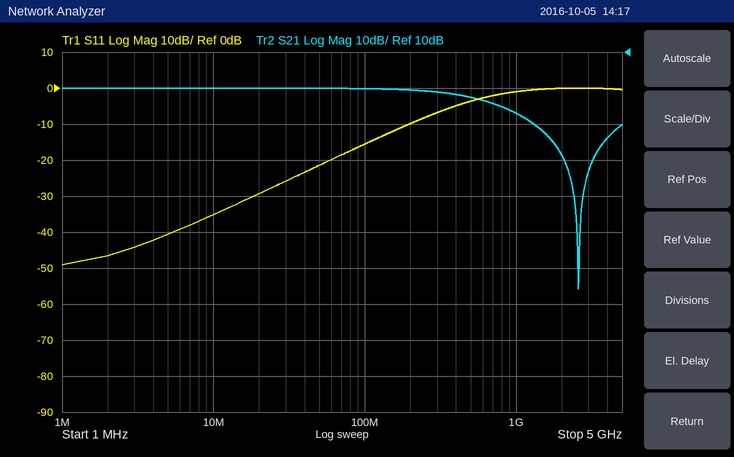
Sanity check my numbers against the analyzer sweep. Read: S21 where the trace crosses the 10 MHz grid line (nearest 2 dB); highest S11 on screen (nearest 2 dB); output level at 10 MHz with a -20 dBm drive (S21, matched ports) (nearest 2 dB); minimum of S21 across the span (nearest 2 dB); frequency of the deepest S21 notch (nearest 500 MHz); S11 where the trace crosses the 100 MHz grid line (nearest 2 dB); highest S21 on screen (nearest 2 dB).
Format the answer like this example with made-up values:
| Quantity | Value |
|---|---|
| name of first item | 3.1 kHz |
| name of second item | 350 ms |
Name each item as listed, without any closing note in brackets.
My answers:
| Quantity | Value |
|---|---|
| S21 where the trace crosses the 10 MHz grid line | 0 dB |
| highest S11 on screen | 0 dB |
| output level at 10 MHz with a -20 dBm drive (S21, matched ports) | -20 dBm |
| minimum of S21 across the span | -56 dB |
| frequency of the deepest S21 notch | 2.5 GHz |
| S11 where the trace crosses the 100 MHz grid line | -16 dB |
| highest S21 on screen | 0 dB |
